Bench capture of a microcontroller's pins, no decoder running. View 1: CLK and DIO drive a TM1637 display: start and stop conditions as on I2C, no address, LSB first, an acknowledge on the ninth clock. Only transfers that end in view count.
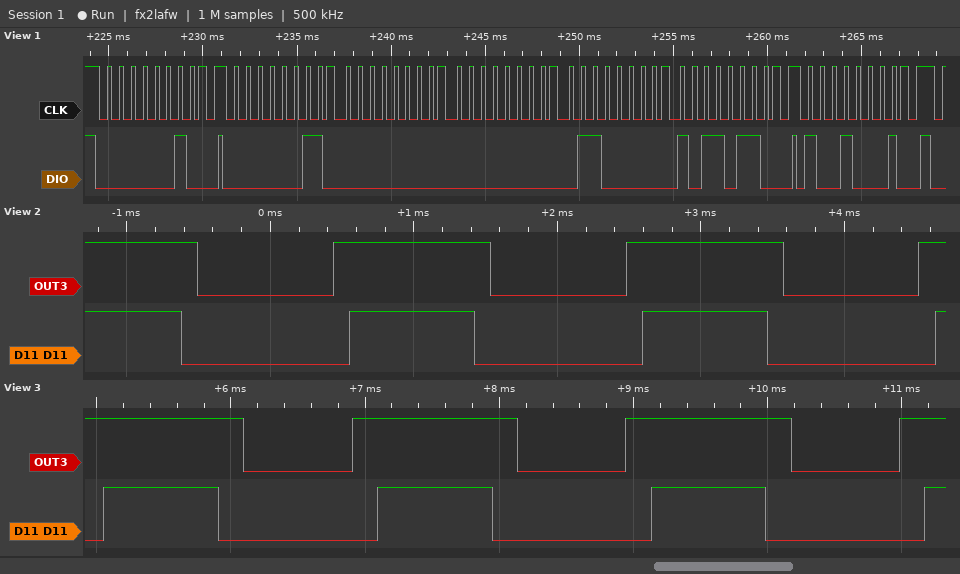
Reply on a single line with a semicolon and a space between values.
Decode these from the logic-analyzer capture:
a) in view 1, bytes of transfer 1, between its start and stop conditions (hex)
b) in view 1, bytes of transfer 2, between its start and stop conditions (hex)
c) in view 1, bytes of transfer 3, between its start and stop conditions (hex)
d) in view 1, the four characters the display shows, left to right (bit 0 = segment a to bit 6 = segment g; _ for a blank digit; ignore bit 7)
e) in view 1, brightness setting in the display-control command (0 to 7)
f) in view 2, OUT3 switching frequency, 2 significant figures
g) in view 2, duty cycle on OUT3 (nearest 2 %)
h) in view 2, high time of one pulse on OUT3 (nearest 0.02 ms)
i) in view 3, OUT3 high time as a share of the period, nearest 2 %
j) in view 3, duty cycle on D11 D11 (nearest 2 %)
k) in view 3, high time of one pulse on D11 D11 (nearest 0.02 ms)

40; C0 00 00 06 6D; 89; __15; 1; 490 Hz; 54 %; 1.10 ms; 60 %; 42 %; 0.86 ms
